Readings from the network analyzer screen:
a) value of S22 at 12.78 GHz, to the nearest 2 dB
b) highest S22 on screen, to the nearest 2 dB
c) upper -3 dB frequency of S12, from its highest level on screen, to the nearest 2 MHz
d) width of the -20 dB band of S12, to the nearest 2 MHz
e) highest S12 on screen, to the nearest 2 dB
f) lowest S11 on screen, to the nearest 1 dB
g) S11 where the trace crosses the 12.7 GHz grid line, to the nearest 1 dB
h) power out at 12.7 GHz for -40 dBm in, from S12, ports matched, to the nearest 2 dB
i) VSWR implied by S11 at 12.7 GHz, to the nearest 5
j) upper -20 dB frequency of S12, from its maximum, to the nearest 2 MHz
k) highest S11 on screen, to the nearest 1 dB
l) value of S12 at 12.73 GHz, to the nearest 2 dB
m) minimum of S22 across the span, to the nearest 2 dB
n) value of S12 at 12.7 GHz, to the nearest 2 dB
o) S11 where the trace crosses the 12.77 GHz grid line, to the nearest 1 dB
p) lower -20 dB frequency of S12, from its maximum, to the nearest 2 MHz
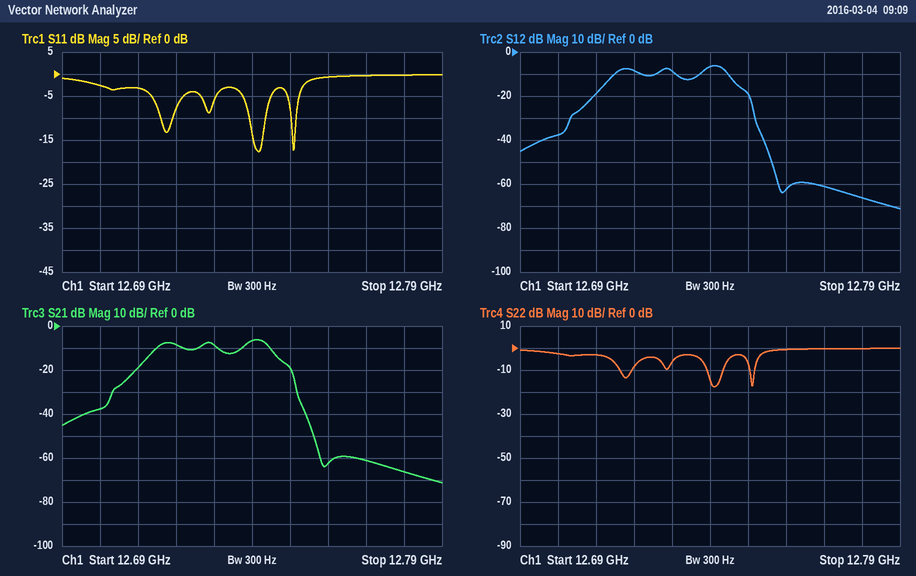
0 dB
0 dB
12.744 GHz
46 MHz
-6 dB
-18 dB
-3 dB
-78 dBm
5
12.752 GHz
0 dB
-8 dB
-18 dB
-38 dB
0 dB
12.706 GHz
